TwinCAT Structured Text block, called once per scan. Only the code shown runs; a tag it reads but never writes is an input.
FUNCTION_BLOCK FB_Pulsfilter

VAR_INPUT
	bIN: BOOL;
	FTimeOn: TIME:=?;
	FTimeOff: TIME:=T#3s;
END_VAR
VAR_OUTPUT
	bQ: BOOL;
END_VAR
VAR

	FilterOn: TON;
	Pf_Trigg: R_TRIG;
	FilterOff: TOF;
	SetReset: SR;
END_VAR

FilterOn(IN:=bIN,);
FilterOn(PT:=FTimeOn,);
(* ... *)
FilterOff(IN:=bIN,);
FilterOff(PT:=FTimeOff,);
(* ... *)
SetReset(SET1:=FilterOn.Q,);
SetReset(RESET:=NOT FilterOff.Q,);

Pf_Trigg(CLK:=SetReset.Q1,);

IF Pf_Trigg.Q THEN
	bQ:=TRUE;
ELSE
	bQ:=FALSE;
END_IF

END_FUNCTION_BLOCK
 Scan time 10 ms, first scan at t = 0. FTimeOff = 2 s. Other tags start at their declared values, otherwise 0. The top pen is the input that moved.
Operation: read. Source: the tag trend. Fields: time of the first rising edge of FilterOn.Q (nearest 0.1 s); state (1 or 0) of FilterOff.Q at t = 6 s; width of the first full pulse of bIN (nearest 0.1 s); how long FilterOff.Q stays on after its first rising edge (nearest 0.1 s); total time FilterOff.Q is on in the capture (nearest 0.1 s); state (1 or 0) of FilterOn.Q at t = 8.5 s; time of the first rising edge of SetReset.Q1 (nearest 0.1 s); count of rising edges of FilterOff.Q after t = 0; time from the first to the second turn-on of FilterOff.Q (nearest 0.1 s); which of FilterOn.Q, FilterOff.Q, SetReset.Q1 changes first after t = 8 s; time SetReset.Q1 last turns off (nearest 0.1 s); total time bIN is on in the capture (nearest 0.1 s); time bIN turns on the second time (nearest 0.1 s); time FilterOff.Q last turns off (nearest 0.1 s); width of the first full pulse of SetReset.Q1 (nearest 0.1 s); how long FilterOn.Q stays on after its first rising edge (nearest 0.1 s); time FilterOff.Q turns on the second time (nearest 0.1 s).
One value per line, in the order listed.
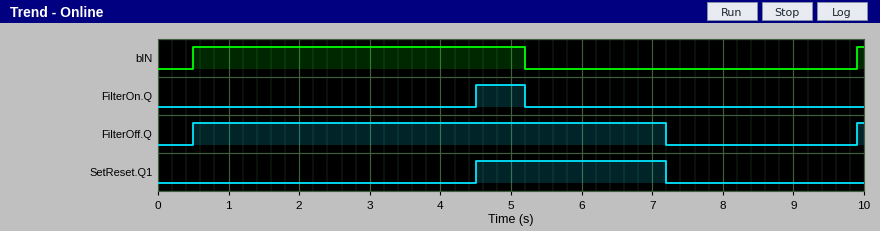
4.5 s
1
4.7 s
6.7 s
6.8 s
0
4.5 s
2
9.4 s
FilterOff.Q
7.2 s
4.8 s
9.9 s
7.2 s
2.7 s
0.7 s
9.9 s
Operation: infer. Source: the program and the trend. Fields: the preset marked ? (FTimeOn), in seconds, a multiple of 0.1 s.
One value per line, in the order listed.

4.0 s
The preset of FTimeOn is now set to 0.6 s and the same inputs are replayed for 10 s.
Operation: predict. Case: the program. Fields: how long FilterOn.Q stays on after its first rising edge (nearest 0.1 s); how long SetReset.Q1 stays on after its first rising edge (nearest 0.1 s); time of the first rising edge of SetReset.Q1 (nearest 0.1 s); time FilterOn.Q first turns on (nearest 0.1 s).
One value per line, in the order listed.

4.1 s
6.1 s
1.1 s
1.1 s
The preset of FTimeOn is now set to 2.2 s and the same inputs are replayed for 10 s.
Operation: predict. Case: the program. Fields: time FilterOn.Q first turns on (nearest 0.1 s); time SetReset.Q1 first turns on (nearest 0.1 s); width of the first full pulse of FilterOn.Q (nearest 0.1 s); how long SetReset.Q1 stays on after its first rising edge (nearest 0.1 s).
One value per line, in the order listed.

2.7 s
2.7 s
2.5 s
4.5 s
